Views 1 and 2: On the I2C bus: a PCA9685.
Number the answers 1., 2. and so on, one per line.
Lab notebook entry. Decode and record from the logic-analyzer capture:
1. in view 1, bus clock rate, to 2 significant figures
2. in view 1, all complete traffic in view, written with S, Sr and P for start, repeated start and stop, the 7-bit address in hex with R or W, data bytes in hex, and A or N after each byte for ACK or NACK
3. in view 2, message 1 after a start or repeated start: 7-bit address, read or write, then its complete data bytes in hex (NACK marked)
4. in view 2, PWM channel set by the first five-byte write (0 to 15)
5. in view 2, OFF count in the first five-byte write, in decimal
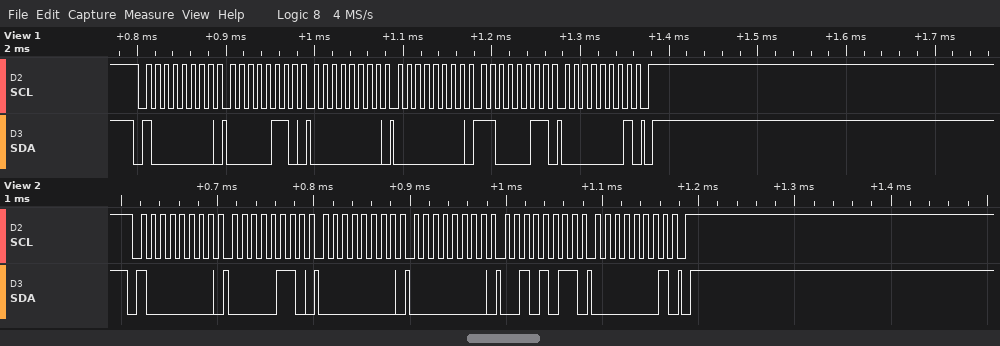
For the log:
1. 100 kHz
2. S 40W A 06 A 00 A 00 A C3 A 01 A P
3. 0x40 write: 06 00 00 2B 01
4. 0
5. 299
